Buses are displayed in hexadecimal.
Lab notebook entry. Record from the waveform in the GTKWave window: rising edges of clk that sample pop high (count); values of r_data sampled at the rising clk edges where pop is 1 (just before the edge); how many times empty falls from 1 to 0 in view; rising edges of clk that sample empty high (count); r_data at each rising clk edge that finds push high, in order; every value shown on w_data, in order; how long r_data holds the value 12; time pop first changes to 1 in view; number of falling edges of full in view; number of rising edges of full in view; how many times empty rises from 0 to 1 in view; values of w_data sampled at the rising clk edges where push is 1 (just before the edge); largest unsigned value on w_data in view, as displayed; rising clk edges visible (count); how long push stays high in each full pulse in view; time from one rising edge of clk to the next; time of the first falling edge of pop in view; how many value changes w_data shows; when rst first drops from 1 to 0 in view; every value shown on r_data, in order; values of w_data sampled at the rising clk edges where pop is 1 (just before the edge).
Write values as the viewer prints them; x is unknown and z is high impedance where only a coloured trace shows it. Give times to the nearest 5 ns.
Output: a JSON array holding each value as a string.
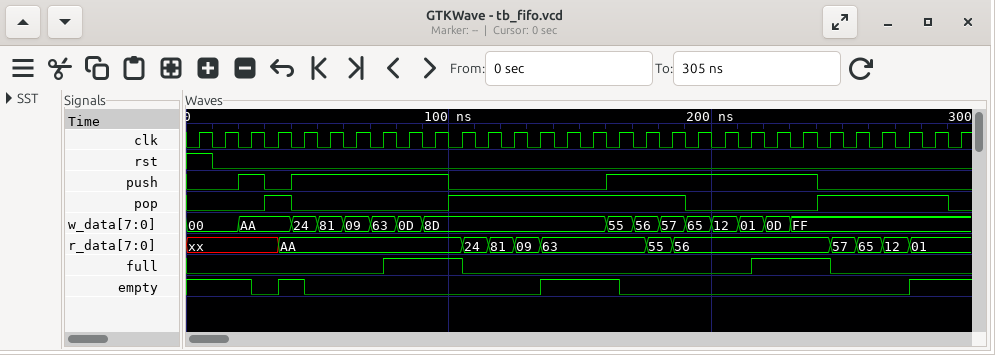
["15", "xx, AA, 24, 81, 09, 63, 63, 63, 63, 55, 56, 57, 65, 12, 01", "3", "9", "xx, AA, AA, AA, AA, AA, AA, 63, 63, 55, 56, 56, 56, 56, 56", "00, AA, 24, 81, 09, 63, 0D, 8D, 55, 56, 57, 65, 12, 01, 0D, FF", "10 ns", "30 ns", "2", "2", "3", "AA, 24, 81, 09, 63, 0D, 8D, 55, 56, 57, 65, 12, 01, 0D, FF", "FF", "30", "10 ns, 60 ns, 80 ns", "10 ns", "40 ns", "15", "10 ns", "xx, AA, 24, 81, 09, 63, 55, 56, 57, 65, 12, 01", "AA, 8D, 8D, 8D, 8D, 8D, 8D, 55, 56, 57, FF, FF, FF, FF, FF"]
